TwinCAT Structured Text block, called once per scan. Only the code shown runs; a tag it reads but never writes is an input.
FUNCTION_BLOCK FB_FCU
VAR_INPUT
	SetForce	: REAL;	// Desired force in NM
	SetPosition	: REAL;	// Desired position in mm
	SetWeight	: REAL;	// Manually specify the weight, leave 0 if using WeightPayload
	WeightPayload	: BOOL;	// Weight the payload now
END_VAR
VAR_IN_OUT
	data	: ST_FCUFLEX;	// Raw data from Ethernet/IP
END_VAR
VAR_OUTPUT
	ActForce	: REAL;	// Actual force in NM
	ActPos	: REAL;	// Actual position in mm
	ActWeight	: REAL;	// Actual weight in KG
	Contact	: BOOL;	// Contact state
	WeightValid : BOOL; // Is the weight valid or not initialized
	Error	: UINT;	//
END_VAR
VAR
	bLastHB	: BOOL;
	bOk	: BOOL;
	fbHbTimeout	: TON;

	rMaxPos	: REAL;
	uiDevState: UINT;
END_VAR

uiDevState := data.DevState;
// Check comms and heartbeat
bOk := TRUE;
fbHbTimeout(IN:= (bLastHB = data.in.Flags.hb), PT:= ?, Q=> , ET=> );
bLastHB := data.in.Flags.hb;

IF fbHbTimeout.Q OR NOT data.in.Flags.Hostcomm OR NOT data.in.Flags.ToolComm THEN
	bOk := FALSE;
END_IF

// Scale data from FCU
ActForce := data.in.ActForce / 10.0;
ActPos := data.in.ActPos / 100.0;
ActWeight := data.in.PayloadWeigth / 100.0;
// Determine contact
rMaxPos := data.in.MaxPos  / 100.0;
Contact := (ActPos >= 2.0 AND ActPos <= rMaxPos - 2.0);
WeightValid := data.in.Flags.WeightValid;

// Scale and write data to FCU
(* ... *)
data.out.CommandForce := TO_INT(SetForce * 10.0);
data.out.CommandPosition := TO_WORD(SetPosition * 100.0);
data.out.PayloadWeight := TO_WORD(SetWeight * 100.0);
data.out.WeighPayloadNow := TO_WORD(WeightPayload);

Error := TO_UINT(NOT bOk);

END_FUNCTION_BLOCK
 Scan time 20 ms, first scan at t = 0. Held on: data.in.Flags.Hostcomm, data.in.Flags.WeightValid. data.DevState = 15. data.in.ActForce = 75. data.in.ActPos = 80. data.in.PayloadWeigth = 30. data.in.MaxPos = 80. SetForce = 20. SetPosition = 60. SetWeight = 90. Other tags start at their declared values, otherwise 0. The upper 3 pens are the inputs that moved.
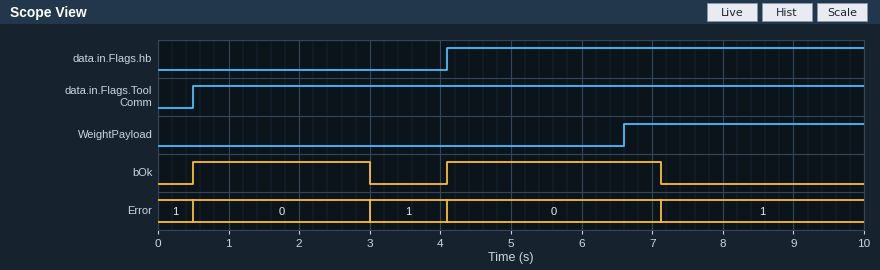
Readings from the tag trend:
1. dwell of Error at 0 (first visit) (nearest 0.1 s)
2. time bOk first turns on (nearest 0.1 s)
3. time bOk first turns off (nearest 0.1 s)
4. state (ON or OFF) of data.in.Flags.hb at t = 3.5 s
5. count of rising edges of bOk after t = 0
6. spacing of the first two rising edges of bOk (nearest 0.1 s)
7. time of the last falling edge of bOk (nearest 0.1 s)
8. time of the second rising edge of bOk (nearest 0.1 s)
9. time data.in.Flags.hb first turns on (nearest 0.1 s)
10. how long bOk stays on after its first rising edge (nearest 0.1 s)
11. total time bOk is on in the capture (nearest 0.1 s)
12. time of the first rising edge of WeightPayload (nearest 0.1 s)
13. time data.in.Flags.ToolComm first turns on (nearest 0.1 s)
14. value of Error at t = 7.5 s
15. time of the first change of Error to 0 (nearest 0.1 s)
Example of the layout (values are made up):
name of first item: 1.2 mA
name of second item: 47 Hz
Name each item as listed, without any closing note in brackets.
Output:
dwell of Error at 0 (first visit): 2.5 s
time bOk first turns on: 0.5 s
time bOk first turns off: 3.0 s
state (ON or OFF) of data.in.Flags.hb at t = 3.5 s: OFF
count of rising edges of bOk after t = 0: 2
spacing of the first two rising edges of bOk: 3.6 s
time of the last falling edge of bOk: 7.1 s
time of the second rising edge of bOk: 4.1 s
time data.in.Flags.hb first turns on: 4.1 s
how long bOk stays on after its first rising edge: 2.5 s
total time bOk is on in the capture: 5.5 s
time of the first rising edge of WeightPayload: 6.6 s
time data.in.Flags.ToolComm first turns on: 0.5 s
value of Error at t = 7.5 s: 1
time of the first change of Error to 0: 0.5 s
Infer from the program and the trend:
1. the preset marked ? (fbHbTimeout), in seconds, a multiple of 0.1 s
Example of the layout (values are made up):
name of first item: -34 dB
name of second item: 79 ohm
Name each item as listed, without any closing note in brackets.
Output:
the preset marked ? (fbHbTimeout), in seconds, a multiple of 0.1 s: 3.0 s
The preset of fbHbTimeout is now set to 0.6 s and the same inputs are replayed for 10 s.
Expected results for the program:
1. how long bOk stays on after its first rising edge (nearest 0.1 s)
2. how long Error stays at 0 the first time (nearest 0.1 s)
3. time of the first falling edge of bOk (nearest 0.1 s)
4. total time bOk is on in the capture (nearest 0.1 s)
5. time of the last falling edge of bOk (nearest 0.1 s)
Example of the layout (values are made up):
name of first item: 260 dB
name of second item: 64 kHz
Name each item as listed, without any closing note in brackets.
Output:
how long bOk stays on after its first rising edge: 0.1 s
how long Error stays at 0 the first time: 0.1 s
time of the first falling edge of bOk: 0.6 s
total time bOk is on in the capture: 0.7 s
time of the last falling edge of bOk: 4.7 s
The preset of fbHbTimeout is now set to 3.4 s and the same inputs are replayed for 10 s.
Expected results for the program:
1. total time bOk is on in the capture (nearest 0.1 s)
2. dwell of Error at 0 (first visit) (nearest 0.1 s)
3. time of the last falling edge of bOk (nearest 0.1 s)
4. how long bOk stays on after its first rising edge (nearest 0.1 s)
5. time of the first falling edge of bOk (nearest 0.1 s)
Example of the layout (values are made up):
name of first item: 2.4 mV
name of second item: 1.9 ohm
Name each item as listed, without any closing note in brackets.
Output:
total time bOk is on in the capture: 6.3 s
dwell of Error at 0 (first visit): 2.9 s
time of the last falling edge of bOk: 7.5 s
how long bOk stays on after its first rising edge: 2.9 s
time of the first falling edge of bOk: 3.4 s
